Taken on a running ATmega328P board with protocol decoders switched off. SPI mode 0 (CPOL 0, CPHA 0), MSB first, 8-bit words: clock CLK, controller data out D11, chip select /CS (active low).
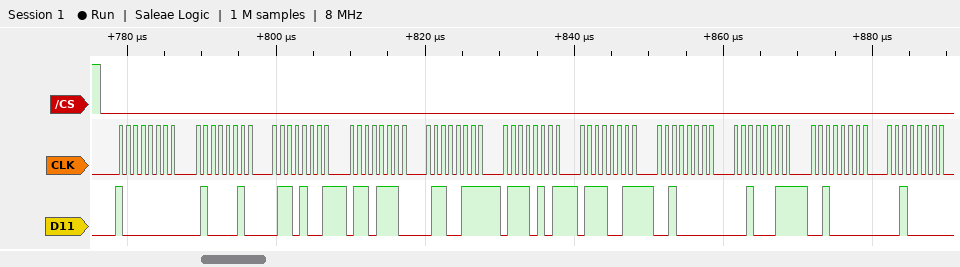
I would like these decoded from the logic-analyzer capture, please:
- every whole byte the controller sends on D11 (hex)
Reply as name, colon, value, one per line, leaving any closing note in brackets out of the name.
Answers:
every whole byte the controller sends on D11: 80 42 69 6E 67 75 73 20 23 20 20
